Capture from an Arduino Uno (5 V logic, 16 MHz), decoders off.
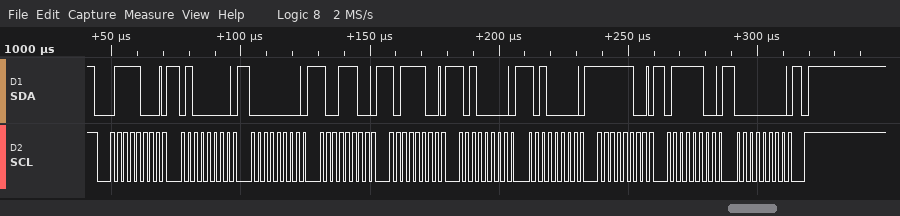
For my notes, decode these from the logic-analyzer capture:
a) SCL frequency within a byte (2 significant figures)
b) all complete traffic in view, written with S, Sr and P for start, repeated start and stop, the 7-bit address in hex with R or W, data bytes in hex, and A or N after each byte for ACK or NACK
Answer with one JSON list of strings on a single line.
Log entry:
["400 kHz", "S 3CW A 40 A 00 A 9C A BC A A0 A A0 A FC A 7C A 00 A P"]
